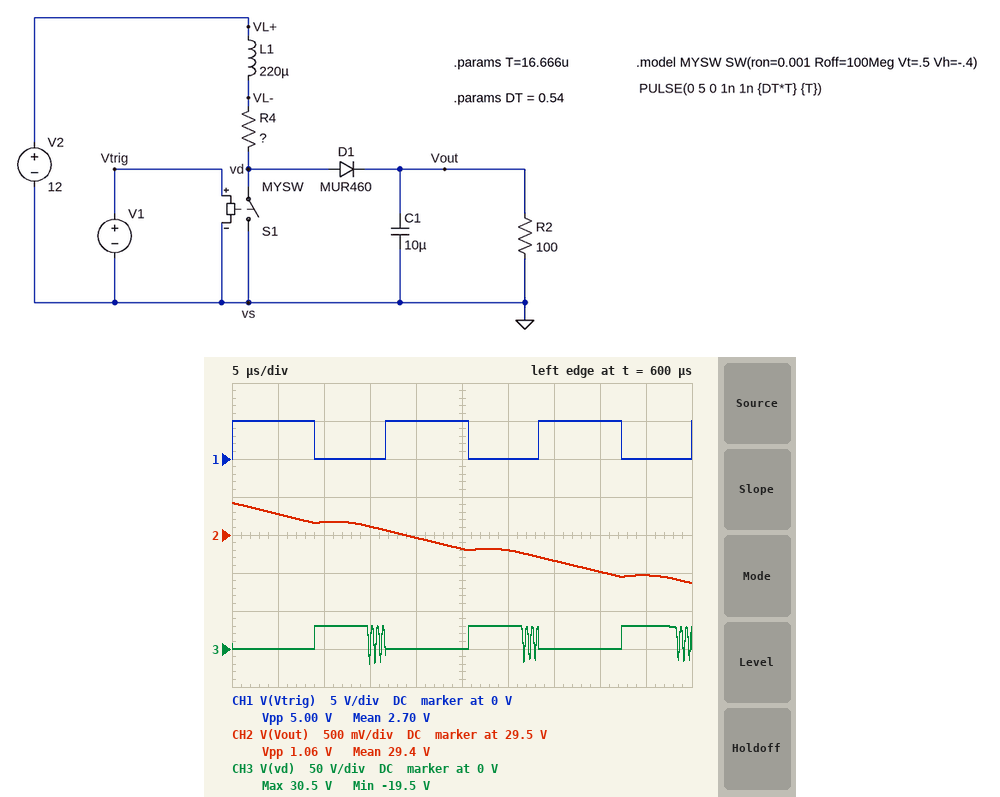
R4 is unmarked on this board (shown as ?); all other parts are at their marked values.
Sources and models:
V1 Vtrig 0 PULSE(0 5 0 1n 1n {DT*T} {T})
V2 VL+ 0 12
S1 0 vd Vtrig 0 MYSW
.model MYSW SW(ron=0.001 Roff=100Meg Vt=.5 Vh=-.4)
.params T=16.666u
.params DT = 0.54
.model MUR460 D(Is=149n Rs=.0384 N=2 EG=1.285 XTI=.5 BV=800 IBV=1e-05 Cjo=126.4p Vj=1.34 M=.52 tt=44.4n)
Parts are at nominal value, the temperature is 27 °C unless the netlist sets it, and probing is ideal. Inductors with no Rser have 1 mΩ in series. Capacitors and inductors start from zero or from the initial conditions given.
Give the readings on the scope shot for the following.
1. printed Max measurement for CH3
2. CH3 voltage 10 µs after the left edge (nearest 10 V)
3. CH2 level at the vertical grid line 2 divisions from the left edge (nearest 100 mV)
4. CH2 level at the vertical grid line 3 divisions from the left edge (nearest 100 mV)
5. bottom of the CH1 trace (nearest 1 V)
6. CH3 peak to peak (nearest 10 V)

30.5 V
30 V
29.7 V
29.6 V
0 V
50 V
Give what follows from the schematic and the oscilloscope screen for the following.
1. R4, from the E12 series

0.68 Ω
